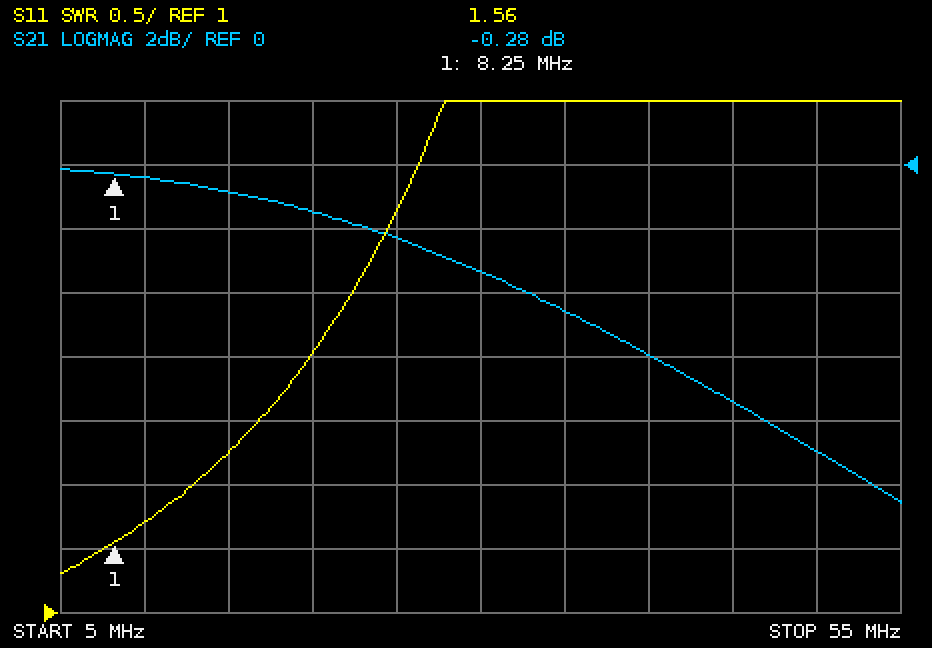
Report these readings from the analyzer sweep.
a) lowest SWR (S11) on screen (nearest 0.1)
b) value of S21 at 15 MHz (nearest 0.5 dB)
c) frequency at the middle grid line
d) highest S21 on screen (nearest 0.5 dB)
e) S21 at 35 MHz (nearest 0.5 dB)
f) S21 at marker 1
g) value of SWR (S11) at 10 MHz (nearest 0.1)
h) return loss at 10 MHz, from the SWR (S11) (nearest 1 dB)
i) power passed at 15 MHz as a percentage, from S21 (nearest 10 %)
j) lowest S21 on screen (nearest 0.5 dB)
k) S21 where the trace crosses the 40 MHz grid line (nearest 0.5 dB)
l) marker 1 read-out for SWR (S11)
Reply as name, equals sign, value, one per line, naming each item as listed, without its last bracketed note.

lowest SWR (S11) on screen = 1.3
value of S21 at 15 MHz = -1.0 dB
frequency at the middle grid line = 30 MHz
highest S21 on screen = 0.0 dB
S21 at 35 MHz = -4.5 dB
S21 at marker 1 = -0.28 dB
value of SWR (S11) at 10 MHz = 1.7
return loss at 10 MHz, from the SWR (S11) = 12 dB
power passed at 15 MHz as a percentage, from S21 = 80 %
lowest S21 on screen = -10.5 dB
S21 where the trace crosses the 40 MHz grid line = -6.0 dB
marker 1 read-out for SWR = 1.56
